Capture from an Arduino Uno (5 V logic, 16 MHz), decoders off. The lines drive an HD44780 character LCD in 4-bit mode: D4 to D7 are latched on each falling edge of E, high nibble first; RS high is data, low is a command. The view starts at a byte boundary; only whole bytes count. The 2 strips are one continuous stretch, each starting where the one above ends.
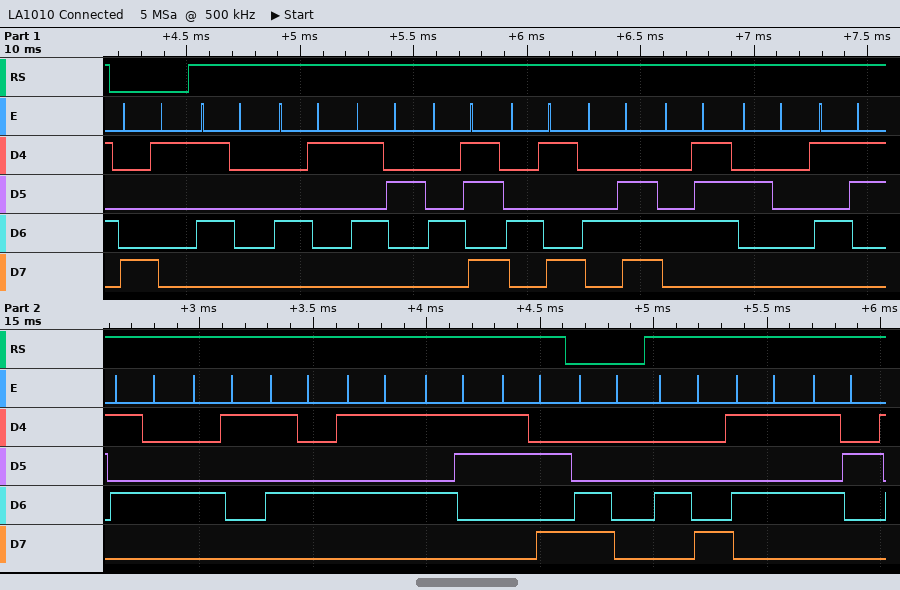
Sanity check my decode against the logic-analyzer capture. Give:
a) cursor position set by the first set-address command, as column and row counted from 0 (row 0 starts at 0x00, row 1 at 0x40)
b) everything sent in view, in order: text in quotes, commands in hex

column 1, row 0
0x81 "PARKING STATUS:" 0xC0 "HUR"
